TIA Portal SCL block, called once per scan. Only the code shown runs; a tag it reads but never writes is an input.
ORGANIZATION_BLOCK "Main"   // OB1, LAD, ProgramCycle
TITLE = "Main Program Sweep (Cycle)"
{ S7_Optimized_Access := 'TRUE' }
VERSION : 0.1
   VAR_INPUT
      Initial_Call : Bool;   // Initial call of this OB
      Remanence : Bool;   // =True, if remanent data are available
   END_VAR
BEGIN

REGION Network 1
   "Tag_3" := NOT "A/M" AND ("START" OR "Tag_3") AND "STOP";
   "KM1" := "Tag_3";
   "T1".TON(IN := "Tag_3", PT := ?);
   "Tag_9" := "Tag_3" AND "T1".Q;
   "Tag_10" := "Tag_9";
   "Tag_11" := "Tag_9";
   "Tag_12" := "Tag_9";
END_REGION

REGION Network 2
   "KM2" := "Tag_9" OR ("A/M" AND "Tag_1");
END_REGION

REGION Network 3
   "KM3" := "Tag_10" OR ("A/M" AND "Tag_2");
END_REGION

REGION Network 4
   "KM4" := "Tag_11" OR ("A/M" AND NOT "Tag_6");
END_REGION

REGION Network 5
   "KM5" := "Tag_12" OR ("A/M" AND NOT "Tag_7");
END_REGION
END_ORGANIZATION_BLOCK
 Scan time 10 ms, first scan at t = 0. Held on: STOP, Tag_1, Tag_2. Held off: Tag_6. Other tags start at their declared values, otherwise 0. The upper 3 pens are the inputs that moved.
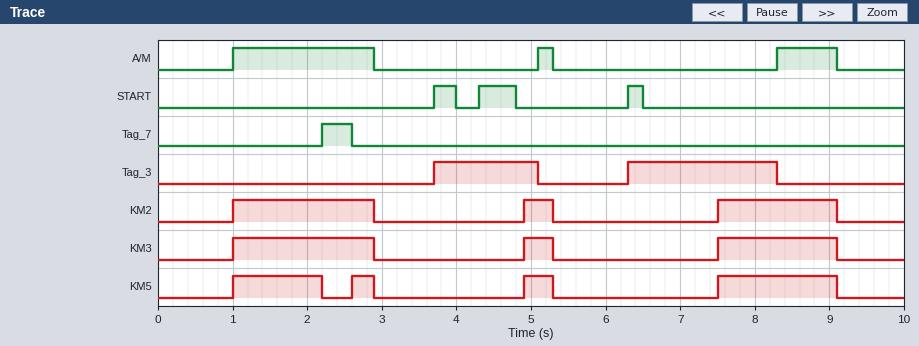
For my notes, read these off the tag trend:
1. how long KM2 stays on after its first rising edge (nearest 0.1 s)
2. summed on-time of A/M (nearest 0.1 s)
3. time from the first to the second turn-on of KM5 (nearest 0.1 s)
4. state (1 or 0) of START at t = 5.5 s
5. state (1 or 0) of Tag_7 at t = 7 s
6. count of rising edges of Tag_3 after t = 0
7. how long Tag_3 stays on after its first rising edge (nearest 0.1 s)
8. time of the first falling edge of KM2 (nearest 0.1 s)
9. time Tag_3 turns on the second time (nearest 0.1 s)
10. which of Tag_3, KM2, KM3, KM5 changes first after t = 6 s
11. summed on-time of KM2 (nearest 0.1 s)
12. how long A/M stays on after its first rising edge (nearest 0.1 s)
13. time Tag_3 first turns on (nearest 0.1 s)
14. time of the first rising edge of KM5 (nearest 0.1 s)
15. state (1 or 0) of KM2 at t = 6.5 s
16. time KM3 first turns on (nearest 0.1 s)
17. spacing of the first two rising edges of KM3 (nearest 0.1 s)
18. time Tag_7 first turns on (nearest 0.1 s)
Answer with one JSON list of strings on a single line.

["1.9 s", "2.9 s", "1.6 s", "0", "0", "2", "1.4 s", "2.9 s", "6.3 s", "Tag_3", "3.9 s", "1.9 s", "3.7 s", "1.0 s", "0", "1.0 s", "3.9 s", "2.2 s"]
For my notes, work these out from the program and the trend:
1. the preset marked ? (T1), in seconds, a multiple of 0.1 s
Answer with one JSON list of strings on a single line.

["1.2 s"]
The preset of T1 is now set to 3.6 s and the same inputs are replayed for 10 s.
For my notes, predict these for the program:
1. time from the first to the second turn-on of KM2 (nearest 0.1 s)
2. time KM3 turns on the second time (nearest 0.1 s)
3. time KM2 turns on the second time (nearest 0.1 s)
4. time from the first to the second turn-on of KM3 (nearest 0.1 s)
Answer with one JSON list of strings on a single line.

["4.1 s", "5.1 s", "5.1 s", "4.1 s"]
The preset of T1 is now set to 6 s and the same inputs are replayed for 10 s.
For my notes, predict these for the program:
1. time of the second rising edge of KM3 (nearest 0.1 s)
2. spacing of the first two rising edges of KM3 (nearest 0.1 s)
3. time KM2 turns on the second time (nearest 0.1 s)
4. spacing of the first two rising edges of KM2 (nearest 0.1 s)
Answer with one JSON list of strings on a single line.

["5.1 s", "4.1 s", "5.1 s", "4.1 s"]
